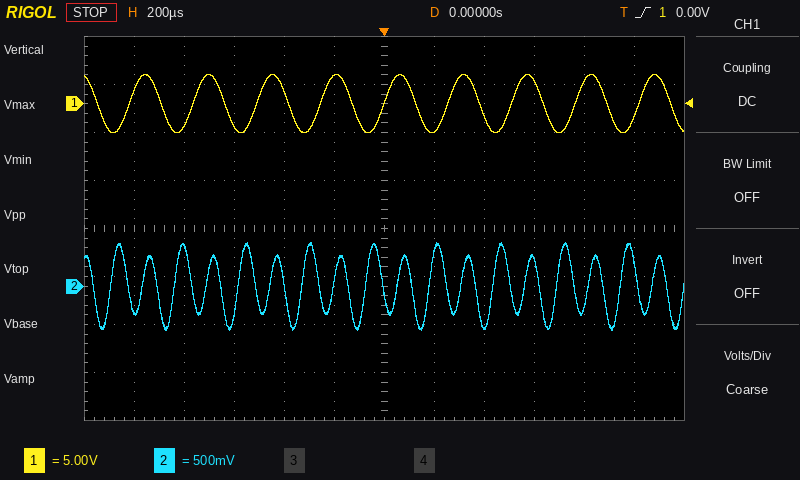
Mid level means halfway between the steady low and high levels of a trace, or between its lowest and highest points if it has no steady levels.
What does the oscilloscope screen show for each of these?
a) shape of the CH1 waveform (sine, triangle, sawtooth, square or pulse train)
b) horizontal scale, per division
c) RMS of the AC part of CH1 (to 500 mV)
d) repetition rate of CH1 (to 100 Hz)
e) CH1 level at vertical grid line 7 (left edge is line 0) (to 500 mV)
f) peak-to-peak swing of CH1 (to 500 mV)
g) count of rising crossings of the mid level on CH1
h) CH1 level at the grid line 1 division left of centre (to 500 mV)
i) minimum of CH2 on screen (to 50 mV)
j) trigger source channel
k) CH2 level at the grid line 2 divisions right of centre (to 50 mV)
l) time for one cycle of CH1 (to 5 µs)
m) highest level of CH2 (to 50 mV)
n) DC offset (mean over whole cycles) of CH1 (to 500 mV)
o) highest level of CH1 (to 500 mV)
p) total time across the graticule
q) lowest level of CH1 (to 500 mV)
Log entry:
sine
200 µs
2.0 V
3.9 kHz
-3.0 V
6.0 V
9
3.0 V
-450 mV
CH1
-400 mV
255 µs
450 mV
0.0 V
3.0 V
2.4 ms
-3.0 V
